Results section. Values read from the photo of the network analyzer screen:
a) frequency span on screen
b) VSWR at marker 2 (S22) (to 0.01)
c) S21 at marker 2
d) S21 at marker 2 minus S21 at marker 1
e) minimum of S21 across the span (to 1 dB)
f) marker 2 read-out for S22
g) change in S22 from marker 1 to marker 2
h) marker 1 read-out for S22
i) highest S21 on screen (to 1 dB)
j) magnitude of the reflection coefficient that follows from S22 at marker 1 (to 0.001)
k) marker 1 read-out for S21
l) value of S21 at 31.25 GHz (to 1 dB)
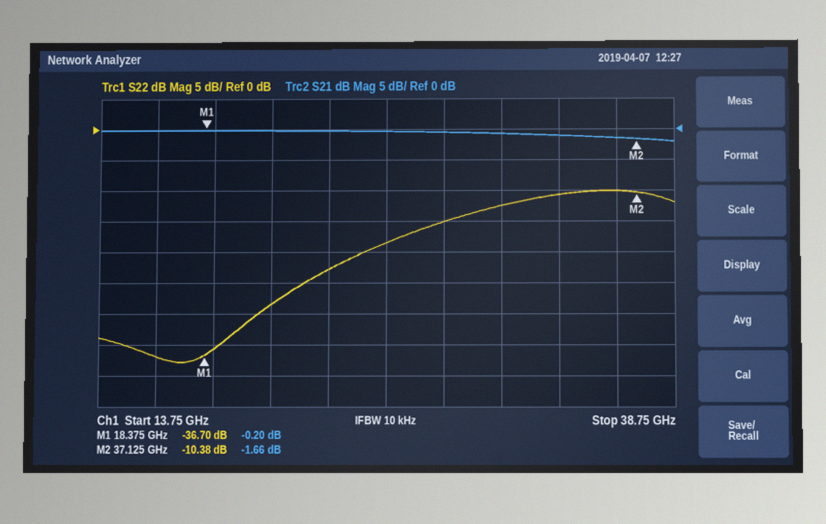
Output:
25 GHz
1.87
-1.66 dB
-1.46 dB
-2 dB
-10.38 dB
26.32 dB
-36.70 dB
0 dB
0.015
-0.20 dB
-1 dB
